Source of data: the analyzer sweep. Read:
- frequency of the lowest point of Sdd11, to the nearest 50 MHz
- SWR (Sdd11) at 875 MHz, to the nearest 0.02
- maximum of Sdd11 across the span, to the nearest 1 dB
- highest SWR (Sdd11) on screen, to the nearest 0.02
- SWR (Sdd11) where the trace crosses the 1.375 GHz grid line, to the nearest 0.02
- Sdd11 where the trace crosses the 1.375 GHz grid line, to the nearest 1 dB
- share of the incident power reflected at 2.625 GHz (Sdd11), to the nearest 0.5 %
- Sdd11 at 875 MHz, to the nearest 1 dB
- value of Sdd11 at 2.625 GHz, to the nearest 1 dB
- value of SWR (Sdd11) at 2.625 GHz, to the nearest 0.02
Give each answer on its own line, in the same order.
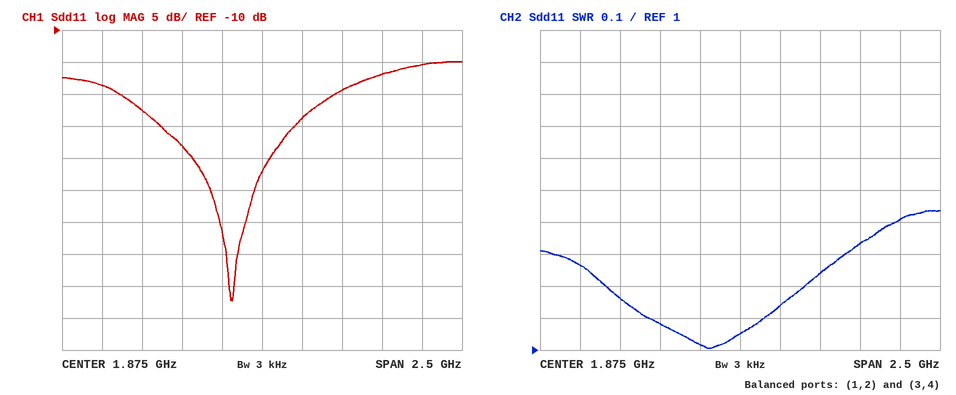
1.70 GHz
1.26
-15 dB
1.44
1.08
-28 dB
2.0 %
-19 dB
-17 dB
1.34
